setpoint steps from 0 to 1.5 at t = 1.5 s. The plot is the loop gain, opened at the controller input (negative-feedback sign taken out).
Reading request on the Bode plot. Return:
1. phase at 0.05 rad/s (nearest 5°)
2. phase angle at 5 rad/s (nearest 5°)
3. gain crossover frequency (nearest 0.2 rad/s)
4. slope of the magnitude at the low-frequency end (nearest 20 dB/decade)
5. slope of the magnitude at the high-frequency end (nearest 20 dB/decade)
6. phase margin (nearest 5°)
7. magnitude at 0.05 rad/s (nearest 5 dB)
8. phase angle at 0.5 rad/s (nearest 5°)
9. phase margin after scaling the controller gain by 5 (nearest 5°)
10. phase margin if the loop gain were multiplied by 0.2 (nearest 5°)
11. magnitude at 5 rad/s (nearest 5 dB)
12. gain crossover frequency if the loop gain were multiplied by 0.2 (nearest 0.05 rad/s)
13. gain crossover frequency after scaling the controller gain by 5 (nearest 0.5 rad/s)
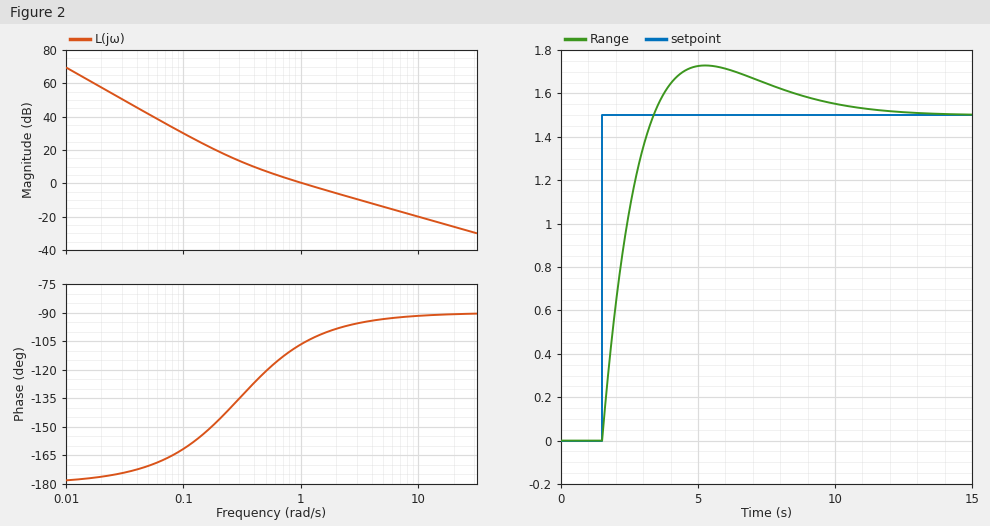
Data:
-170°
-95°
1.0 rad/s
-40 dB/decade
-20 dB/decade
75°
40 dB
-120°
85°
45°
-15 dB
0.30 rad/s
5.0 rad/s
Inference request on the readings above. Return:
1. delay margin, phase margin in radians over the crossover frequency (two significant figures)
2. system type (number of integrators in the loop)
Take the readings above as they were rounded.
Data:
1.3 s
2
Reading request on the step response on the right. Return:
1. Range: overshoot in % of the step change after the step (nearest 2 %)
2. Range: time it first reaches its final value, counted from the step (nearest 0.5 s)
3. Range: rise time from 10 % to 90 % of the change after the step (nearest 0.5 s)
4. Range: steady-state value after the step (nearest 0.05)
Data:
16 %
2.0 s
1.5 s
1.50
